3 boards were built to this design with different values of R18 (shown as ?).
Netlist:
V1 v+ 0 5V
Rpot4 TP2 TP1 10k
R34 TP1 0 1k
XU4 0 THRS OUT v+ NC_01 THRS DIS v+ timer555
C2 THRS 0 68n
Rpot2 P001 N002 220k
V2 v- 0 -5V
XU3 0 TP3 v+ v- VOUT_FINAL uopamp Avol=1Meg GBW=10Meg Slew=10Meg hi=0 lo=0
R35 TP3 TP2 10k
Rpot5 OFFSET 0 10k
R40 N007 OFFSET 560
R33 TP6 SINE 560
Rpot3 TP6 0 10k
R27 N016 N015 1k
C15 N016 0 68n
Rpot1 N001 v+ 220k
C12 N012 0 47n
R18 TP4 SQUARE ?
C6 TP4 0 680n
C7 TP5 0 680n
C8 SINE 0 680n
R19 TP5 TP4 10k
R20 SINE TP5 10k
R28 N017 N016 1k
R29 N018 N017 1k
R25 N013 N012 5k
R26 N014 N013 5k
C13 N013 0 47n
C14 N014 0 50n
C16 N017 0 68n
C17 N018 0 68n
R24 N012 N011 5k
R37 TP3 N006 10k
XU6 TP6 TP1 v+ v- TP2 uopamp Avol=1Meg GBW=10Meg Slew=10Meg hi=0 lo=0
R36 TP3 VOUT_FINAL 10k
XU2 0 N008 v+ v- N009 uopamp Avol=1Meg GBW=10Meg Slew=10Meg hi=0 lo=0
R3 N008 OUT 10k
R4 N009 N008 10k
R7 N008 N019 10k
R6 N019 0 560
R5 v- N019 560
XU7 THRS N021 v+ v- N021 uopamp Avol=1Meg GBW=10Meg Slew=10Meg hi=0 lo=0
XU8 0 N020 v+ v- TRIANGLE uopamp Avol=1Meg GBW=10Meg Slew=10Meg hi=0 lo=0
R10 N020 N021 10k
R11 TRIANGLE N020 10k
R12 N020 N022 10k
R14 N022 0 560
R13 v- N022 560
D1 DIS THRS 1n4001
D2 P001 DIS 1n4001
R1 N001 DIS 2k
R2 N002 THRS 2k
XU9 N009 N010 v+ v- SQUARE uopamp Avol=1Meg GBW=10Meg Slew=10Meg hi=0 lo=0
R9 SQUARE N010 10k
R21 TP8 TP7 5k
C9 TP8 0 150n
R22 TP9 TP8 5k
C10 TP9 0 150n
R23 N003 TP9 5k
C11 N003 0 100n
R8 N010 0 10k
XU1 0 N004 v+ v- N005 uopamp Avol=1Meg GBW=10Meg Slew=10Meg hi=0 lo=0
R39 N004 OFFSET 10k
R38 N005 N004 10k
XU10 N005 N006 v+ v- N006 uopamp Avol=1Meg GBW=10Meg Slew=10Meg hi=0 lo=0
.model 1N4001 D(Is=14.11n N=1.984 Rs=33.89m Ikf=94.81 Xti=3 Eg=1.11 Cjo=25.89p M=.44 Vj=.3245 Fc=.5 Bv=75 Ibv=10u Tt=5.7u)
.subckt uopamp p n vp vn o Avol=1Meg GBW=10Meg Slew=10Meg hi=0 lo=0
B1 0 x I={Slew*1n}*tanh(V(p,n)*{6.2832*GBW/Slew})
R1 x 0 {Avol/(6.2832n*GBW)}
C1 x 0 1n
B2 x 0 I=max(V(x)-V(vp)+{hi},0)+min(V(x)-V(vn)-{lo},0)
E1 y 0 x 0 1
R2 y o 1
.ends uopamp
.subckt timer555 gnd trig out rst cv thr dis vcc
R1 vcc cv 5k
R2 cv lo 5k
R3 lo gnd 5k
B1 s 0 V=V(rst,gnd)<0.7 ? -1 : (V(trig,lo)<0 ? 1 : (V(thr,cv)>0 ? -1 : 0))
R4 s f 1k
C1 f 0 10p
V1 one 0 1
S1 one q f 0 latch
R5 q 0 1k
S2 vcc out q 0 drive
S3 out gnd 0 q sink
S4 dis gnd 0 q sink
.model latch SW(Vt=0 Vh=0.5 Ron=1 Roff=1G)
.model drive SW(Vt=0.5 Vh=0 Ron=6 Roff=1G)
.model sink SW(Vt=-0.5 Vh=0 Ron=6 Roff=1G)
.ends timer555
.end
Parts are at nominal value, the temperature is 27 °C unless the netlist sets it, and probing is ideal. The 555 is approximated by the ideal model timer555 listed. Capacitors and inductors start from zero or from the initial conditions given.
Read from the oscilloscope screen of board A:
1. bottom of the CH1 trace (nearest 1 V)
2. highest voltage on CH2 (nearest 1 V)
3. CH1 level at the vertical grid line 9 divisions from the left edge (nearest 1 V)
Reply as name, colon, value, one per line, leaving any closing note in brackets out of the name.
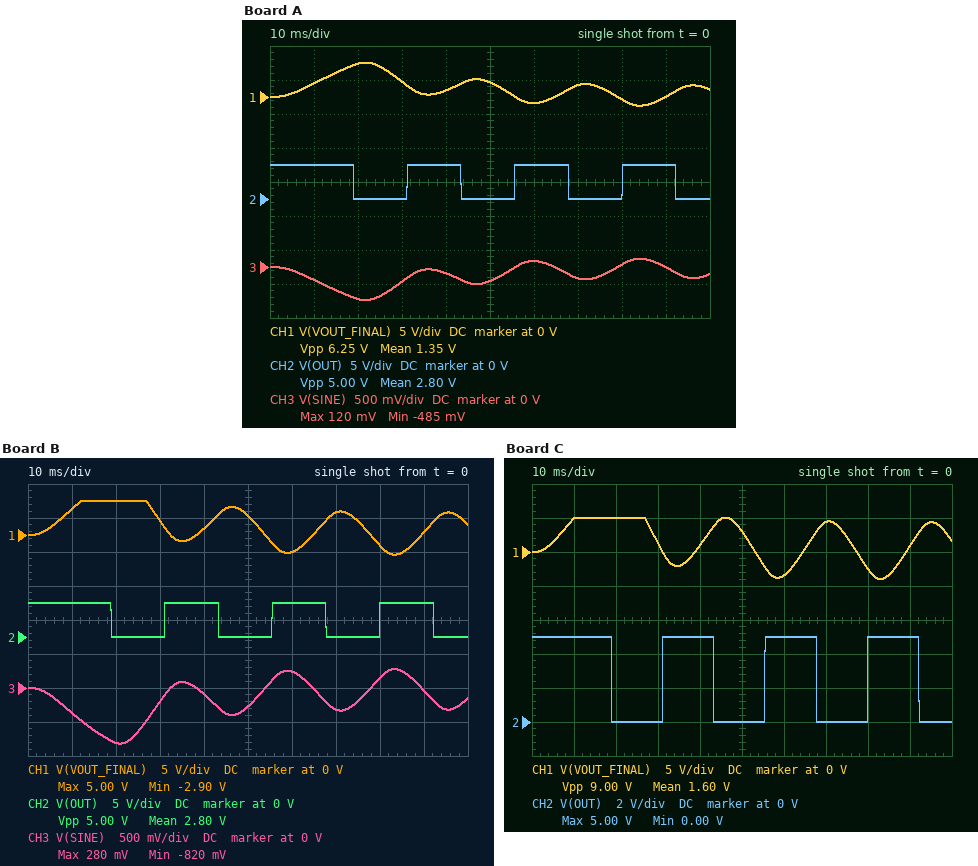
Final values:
bottom of the CH1 trace: -1 V
highest voltage on CH2: 5 V
CH1 level at the vertical grid line 9 divisions from the left edge: 0 V
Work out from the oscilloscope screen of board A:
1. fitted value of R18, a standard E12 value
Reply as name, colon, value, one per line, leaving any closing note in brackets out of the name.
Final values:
fitted value of R18, a standard E12 value: 27 kΩ
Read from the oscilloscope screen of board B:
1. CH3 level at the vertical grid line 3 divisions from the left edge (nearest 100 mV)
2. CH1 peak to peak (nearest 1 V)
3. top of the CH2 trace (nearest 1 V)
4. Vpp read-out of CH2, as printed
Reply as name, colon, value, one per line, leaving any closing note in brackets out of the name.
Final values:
CH3 level at the vertical grid line 3 divisions from the left edge: -200 mV
CH1 peak to peak: 8 V
top of the CH2 trace: 5 V
Vpp read-out of CH2, as printed: 5.00 V
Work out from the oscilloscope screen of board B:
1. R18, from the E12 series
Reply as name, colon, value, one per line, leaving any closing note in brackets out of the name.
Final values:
R18, from the E12 series: 12 kΩ
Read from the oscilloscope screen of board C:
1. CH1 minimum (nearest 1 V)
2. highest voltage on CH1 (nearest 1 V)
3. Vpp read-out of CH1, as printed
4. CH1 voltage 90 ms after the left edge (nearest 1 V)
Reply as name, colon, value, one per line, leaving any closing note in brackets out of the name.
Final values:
CH1 minimum: -4 V
highest voltage on CH1: 5 V
Vpp read-out of CH1, as printed: 9.00 V
CH1 voltage 90 ms after the left edge: 1 V
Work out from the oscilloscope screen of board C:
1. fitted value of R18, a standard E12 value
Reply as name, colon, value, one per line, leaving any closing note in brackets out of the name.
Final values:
fitted value of R18, a standard E12 value: 8.2 kΩ
